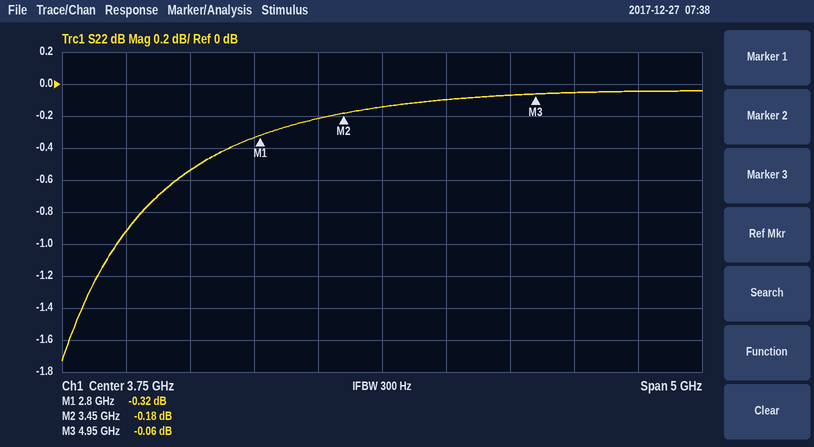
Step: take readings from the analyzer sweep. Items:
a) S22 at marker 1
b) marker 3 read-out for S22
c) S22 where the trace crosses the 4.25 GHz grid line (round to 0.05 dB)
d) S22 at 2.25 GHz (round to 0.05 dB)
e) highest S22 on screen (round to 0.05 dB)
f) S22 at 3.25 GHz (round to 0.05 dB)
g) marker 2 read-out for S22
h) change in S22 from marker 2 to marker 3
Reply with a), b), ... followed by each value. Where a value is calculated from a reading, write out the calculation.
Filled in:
a) -0.32 dB
b) -0.06 dB
c) -0.10 dB
d) -0.55 dB
e) -0.05 dB
f) -0.20 dB
g) -0.18 dB
h) -0.06 − (-0.18) = 0.12 dB
